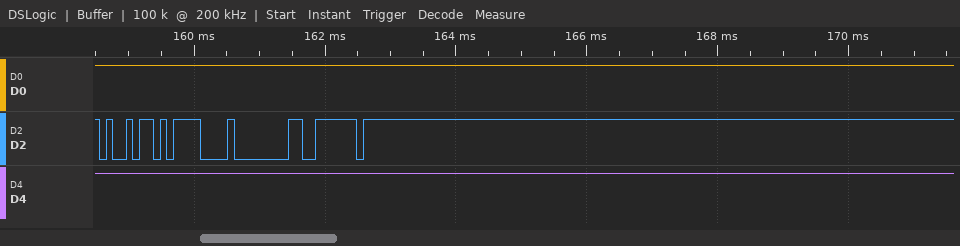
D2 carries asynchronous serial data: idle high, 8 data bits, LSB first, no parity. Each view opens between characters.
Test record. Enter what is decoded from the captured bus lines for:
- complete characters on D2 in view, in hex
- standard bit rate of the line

69, 0F, 80, 7E
9600 baud
